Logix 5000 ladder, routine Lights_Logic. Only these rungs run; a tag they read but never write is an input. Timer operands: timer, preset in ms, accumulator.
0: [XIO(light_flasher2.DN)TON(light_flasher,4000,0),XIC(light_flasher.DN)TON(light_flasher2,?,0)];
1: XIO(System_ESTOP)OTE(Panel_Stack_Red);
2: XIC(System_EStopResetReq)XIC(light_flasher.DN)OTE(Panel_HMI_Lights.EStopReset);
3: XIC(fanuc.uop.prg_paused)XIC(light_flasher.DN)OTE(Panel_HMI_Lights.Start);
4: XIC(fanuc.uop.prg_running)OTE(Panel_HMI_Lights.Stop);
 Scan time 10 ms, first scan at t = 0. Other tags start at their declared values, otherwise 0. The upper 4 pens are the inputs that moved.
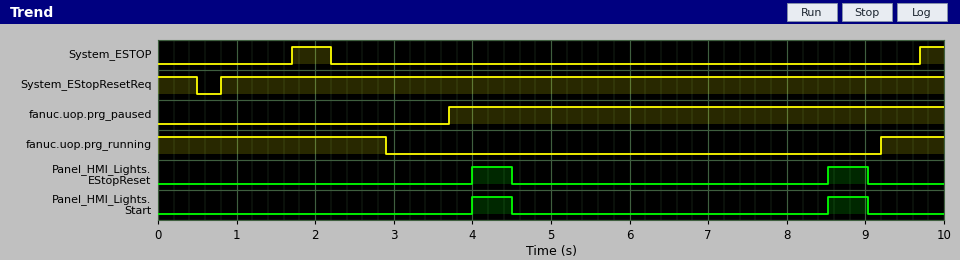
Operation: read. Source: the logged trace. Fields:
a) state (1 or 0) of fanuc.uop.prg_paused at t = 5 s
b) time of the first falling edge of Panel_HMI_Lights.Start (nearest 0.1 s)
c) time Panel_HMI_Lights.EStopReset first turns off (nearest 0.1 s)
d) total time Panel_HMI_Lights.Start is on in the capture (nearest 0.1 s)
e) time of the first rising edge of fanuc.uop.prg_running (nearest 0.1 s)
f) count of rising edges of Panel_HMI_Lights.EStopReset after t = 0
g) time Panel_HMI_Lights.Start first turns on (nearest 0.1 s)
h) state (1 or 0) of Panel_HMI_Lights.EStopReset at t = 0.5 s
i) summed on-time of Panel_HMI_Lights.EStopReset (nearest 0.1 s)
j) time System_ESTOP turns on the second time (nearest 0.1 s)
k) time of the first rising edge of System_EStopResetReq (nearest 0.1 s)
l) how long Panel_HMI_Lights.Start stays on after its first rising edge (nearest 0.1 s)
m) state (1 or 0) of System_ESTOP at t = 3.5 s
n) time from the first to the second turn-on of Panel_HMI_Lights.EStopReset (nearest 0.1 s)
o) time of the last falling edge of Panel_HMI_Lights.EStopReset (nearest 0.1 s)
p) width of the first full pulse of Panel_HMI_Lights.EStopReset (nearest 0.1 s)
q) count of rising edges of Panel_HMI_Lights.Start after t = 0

1
4.5 s
4.5 s
1.0 s
9.2 s
2
4.0 s
0
1.0 s
9.7 s
0.8 s
0.5 s
0
4.5 s
9.0 s
0.5 s
2
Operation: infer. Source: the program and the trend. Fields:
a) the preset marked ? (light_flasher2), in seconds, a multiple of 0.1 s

0.5 s
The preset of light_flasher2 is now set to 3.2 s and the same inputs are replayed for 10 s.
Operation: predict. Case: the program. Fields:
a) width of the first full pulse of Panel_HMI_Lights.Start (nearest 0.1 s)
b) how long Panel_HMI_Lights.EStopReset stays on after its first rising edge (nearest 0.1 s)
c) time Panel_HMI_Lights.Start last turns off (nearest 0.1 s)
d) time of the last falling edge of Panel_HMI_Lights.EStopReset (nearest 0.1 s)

3.2 s
3.2 s
7.2 s
7.2 s
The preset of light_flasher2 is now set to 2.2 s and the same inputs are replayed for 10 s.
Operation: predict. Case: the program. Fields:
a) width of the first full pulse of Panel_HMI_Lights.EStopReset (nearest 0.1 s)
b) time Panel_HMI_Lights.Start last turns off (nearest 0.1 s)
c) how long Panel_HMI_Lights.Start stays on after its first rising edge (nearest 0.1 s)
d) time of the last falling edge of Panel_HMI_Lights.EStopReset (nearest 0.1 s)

2.2 s
6.2 s
2.2 s
6.2 s
